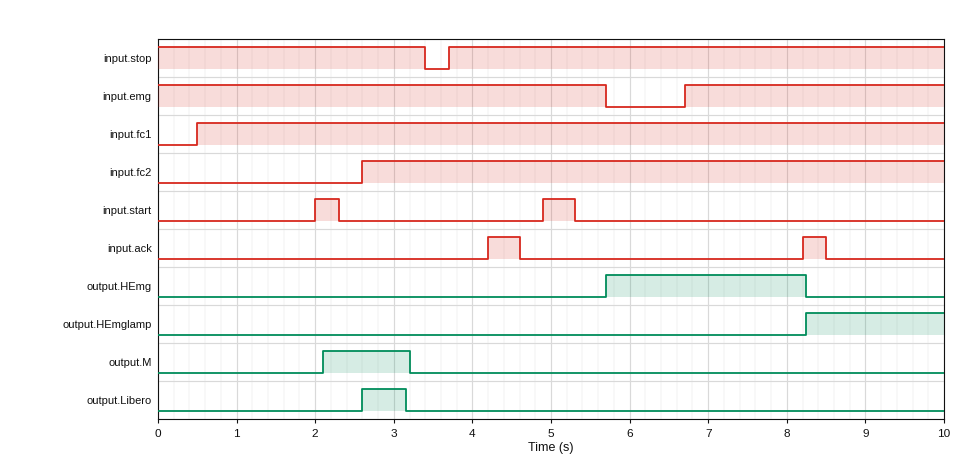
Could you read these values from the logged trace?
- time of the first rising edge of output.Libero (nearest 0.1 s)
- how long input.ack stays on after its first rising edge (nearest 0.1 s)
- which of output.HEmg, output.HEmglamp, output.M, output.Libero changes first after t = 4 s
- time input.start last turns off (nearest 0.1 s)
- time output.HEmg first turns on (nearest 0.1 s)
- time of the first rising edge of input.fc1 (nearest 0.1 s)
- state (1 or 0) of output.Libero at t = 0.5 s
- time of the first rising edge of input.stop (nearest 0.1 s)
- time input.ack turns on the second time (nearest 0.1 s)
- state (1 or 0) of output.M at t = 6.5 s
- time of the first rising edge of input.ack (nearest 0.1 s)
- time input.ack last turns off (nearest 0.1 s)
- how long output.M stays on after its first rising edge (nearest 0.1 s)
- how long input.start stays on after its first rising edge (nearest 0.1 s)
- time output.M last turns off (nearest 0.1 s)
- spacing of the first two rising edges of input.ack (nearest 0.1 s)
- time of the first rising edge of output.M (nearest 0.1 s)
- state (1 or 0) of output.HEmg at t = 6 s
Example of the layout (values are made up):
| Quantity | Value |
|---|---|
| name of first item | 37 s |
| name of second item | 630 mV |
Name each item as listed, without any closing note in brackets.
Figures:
| Quantity | Value |
|---|---|
| time of the first rising edge of output.Libero | 2.6 s |
| how long input.ack stays on after its first rising edge | 0.4 s |
| which of output.HEmg, output.HEmglamp, output.M, output.Libero changes first after t = 4 s | output.HEmg |
| time input.start last turns off | 5.3 s |
| time output.HEmg first turns on | 5.7 s |
| time of the first rising edge of input.fc1 | 0.5 s |
| state (1 or 0) of output.Libero at t = 0.5 s | 0 |
| time of the first rising edge of input.stop | 3.7 s |
| time input.ack turns on the second time | 8.2 s |
| state (1 or 0) of output.M at t = 6.5 s | 0 |
| time of the first rising edge of input.ack | 4.2 s |
| time input.ack last turns off | 8.5 s |
| how long output.M stays on after its first rising edge | 1.1 s |
| how long input.start stays on after its first rising edge | 0.3 s |
| time output.M last turns off | 3.2 s |
| spacing of the first two rising edges of input.ack | 4.0 s |
| time of the first rising edge of output.M | 2.1 s |
| state (1 or 0) of output.HEmg at t = 6 s | 1 |
